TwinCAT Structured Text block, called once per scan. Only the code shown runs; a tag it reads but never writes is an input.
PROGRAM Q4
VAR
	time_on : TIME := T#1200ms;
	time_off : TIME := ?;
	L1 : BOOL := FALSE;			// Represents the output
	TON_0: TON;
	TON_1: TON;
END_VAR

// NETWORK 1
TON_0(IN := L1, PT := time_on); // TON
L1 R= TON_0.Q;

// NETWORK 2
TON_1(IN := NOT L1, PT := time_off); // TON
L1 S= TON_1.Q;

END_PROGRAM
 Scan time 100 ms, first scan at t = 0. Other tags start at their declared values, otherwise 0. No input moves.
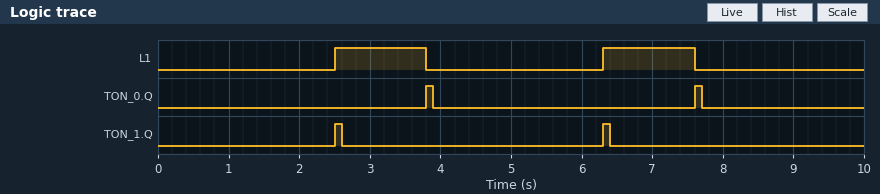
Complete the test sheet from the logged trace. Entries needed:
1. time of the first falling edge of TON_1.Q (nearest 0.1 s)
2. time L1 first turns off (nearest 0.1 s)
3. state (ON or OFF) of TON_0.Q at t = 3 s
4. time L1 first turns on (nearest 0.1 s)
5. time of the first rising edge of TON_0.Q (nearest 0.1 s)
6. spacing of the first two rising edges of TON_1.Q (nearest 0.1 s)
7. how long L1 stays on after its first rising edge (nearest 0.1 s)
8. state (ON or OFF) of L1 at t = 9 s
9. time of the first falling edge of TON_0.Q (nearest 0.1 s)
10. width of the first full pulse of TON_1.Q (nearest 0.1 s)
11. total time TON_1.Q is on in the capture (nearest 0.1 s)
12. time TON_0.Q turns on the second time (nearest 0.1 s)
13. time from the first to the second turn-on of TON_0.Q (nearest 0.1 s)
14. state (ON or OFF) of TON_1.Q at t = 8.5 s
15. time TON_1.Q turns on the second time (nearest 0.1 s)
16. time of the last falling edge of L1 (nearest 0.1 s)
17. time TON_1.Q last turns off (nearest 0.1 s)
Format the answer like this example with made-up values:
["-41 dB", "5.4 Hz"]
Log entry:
["2.6 s", "3.8 s", "OFF", "2.5 s", "3.8 s", "3.8 s", "1.3 s", "OFF", "3.9 s", "0.1 s", "0.2 s", "7.6 s", "3.8 s", "OFF", "6.3 s", "7.6 s", "6.4 s"]
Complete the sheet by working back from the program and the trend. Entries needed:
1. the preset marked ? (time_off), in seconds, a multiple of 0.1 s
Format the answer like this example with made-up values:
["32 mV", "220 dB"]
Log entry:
["2.5 s"]
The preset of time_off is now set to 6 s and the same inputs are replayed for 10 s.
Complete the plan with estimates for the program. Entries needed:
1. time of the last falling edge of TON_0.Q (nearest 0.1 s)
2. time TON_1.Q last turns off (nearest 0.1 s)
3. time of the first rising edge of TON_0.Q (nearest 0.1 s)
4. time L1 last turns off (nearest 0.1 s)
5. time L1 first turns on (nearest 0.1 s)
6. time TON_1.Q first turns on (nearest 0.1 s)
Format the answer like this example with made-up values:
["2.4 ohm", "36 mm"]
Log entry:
["7.4 s", "6.1 s", "7.3 s", "7.3 s", "6.0 s", "6.0 s"]
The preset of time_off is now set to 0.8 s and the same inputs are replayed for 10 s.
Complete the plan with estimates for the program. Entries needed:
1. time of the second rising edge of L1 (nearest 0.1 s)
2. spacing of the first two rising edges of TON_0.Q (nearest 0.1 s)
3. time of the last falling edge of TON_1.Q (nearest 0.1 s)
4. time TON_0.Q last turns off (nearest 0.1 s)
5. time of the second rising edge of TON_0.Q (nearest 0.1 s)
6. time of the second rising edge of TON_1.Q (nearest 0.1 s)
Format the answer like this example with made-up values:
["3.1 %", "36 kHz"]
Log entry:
["2.9 s", "2.1 s", "9.3 s", "8.5 s", "4.2 s", "2.9 s"]
